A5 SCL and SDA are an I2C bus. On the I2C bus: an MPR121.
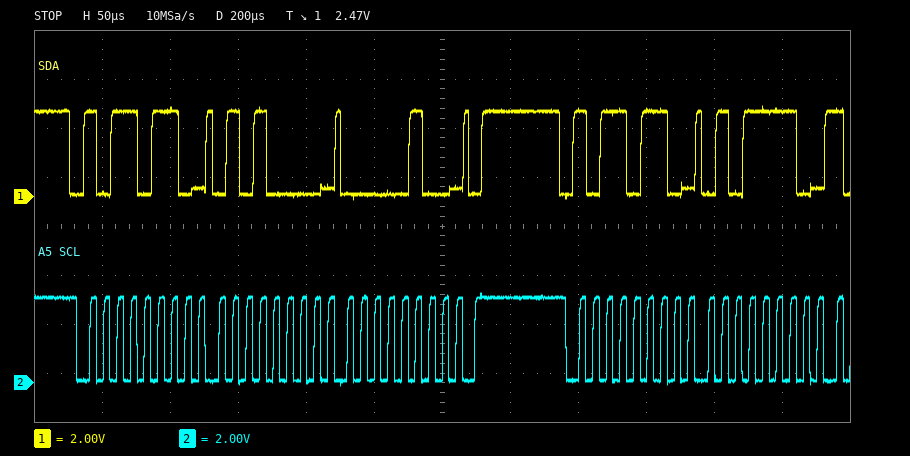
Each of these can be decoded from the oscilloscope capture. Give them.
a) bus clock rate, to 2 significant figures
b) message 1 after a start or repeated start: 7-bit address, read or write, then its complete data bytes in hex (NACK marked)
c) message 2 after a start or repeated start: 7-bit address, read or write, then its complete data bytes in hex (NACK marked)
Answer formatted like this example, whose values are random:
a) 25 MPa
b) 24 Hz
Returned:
a) 100 kHz
b) 0x5B write: 50 04
c) 0x5B write: 5E
